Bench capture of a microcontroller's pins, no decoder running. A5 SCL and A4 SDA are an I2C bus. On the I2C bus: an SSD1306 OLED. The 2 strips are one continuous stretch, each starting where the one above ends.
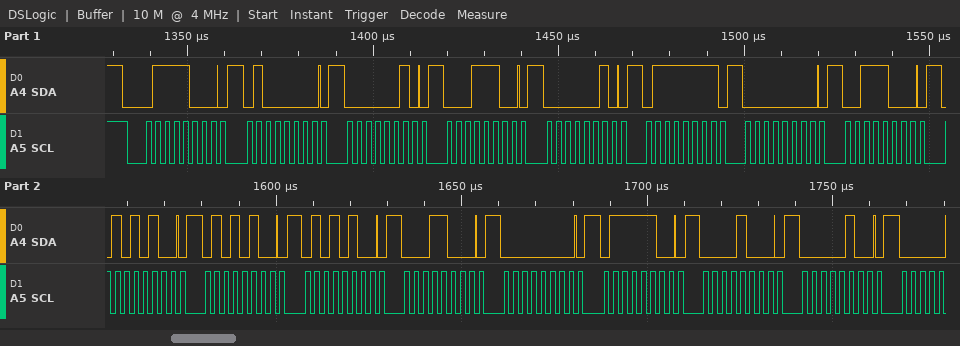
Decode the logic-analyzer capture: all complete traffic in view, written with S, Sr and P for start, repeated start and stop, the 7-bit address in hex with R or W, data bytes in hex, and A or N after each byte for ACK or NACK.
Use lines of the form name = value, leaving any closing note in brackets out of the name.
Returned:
all complete traffic in view, written with S, Sr and P for start, repeated start and stop, the 7-bit address in hex with R or W, data bytes in hex, and A or N after each byte for ACK or NACK = S 3CW A 40 A 02 A 1C A 02 A 7F A 00 A 38 A 54 A 54 A 54 A 18 A 00 A 7C A 08 A 04 A
